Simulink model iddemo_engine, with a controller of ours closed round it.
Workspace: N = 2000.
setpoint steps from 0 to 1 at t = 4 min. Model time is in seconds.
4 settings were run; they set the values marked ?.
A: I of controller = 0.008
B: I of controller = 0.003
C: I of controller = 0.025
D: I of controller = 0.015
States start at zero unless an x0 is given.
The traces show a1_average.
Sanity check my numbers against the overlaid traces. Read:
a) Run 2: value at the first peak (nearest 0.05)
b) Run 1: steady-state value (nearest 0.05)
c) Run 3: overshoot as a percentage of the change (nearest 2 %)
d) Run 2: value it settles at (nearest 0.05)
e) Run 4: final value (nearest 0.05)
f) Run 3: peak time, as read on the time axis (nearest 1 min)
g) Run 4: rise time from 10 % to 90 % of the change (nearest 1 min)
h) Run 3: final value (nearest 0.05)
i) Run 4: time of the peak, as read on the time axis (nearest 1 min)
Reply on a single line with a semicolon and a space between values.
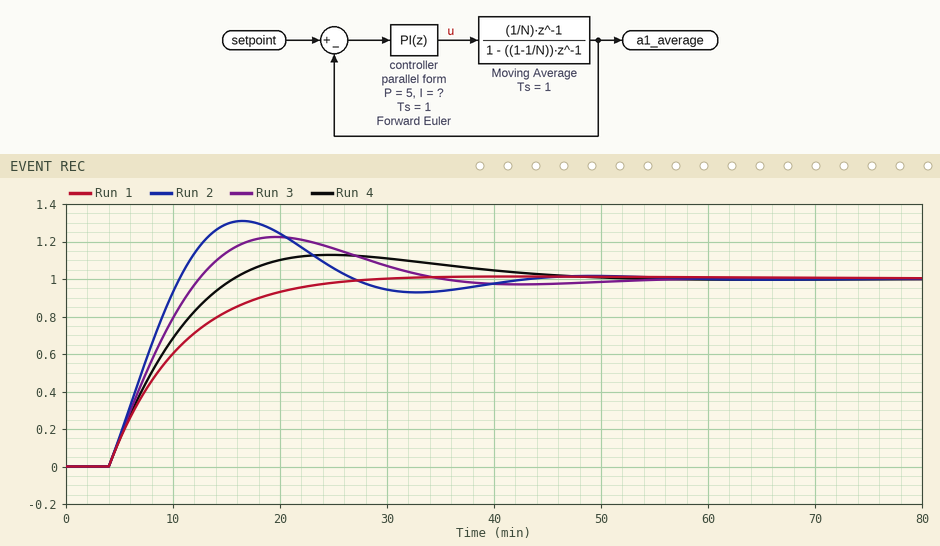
1.30; 1.00; 22 %; 1.00; 1.00; 20 min; 9 min; 1.00; 25 min
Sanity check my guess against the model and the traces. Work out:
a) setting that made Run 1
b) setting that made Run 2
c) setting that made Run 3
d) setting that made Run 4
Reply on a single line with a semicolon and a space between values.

B; C; D; A
